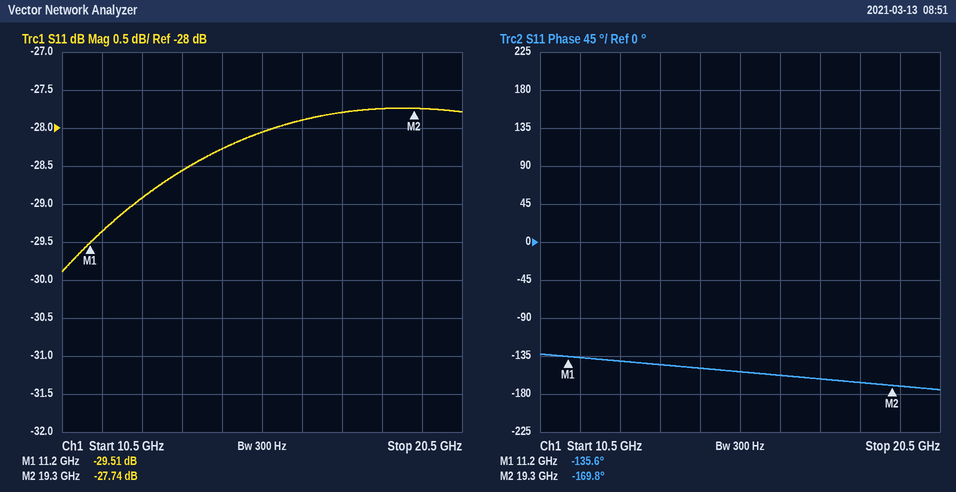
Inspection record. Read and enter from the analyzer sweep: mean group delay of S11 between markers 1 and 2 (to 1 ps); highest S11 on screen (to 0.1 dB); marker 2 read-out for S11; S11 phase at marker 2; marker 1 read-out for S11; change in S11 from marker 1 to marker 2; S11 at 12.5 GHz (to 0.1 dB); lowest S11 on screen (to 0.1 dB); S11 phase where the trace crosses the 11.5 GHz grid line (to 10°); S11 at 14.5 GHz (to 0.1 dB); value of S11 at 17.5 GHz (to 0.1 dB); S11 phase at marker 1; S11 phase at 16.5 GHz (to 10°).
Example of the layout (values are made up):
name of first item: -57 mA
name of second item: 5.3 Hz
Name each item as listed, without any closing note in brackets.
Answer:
mean group delay of S11 between markers 1 and 2: 12 ps
highest S11 on screen: -27.7 dB
marker 2 read-out for S11: -27.74 dB
S11 phase at marker 2: -169.8°
marker 1 read-out for S11: -29.51 dB
change in S11 from marker 1 to marker 2: 1.77 dB
S11 at 12.5 GHz: -28.9 dB
lowest S11 on screen: -29.9 dB
S11 phase where the trace crosses the 11.5 GHz grid line: -140°
S11 at 14.5 GHz: -28.3 dB
value of S11 at 17.5 GHz: -27.8 dB
S11 phase at marker 1: -135.6°
S11 phase at 16.5 GHz: -160°
